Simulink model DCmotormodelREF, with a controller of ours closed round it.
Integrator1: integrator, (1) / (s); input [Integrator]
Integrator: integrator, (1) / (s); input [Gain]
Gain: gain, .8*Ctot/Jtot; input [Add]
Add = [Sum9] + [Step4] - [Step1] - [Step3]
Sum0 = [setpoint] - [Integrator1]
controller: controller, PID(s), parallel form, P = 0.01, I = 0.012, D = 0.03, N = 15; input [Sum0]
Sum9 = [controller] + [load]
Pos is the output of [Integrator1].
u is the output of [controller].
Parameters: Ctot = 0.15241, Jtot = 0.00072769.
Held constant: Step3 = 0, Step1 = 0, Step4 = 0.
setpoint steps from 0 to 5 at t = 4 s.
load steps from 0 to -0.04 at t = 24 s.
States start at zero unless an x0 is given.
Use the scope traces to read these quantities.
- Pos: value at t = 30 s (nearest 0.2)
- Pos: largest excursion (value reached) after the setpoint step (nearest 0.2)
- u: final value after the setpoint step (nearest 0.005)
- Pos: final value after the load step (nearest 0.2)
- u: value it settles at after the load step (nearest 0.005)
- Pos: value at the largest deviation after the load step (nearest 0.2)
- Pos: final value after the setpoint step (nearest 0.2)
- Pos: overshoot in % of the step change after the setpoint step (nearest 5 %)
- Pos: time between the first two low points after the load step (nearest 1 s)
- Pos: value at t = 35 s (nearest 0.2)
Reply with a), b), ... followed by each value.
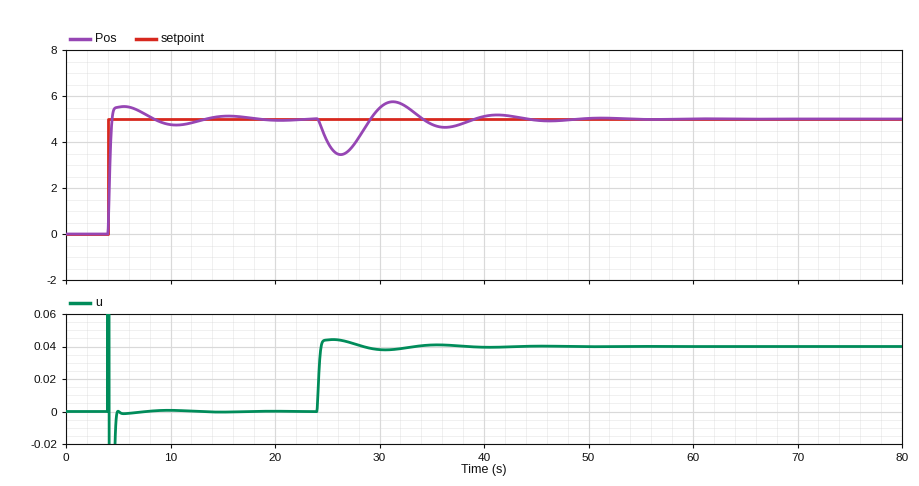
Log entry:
a) 5.4
b) 5.6
c) 0.000
d) 5.0
e) 0.040
f) 3.4
g) 5.0
h) 10 %
i) 10 s
j) 4.8
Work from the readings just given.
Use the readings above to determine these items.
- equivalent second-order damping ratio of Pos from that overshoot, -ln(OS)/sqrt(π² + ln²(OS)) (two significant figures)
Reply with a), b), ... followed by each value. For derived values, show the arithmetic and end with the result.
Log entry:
a) ln(0.1) = -2.303; 2.303 / sqrt(9.870 + 5.302) = 0.59
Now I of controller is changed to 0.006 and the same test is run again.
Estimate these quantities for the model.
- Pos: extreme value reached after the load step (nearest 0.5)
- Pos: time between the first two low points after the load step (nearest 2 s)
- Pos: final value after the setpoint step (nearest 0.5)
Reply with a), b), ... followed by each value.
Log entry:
a) 3.0
b) 14 s
c) 5.0
